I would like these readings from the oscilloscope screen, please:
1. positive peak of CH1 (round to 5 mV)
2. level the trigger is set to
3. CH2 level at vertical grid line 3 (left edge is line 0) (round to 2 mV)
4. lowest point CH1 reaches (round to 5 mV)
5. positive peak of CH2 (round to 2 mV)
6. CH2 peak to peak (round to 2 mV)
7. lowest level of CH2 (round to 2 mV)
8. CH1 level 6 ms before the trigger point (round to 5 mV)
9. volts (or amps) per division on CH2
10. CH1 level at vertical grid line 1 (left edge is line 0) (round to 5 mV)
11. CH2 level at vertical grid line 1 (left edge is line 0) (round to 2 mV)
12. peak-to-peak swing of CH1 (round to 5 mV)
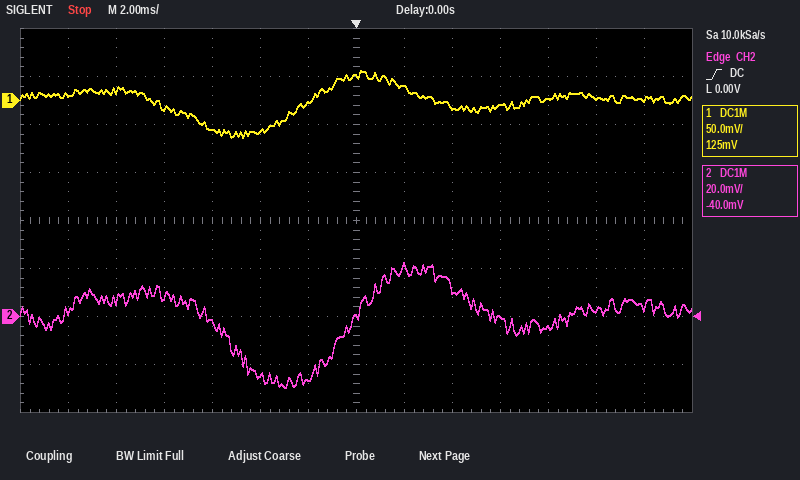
30 mV
0.00 V
8 mV
-40 mV
22 mV
52 mV
-30 mV
-30 mV
20 mV
5 mV
2 mV
70 mV
